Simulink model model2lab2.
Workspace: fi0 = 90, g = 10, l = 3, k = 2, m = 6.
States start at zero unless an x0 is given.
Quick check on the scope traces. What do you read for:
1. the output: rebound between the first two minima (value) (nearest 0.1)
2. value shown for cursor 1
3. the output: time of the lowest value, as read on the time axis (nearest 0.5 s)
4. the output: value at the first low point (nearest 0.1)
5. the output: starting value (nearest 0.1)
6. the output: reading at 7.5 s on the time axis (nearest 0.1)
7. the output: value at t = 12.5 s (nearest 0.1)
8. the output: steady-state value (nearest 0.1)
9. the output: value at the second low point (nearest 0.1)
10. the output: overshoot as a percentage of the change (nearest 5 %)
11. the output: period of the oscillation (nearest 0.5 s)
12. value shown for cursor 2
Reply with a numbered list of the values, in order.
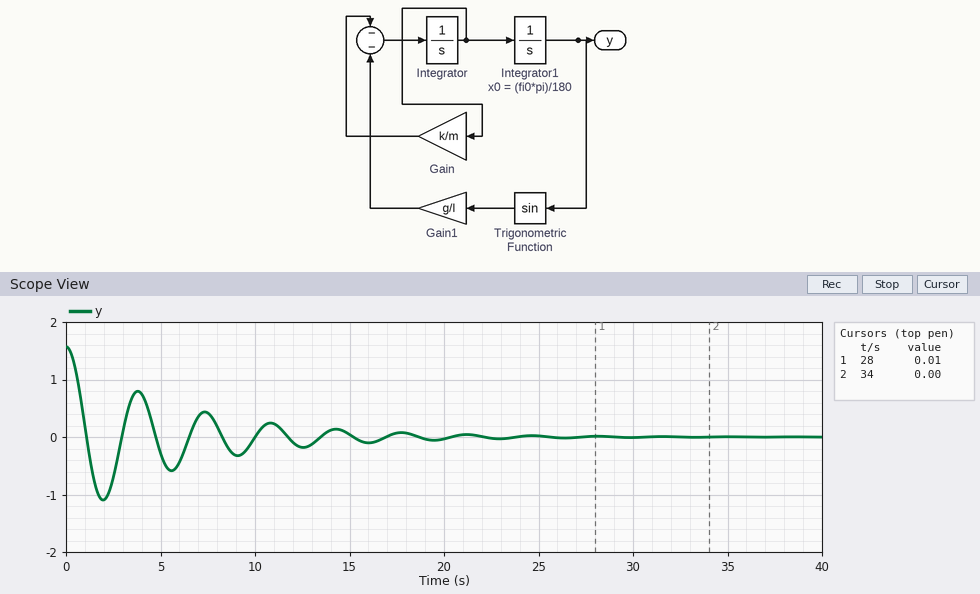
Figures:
1. 0.8
2. 0.01
3. 2.0 s
4. -1.1
5. 1.6
6. 0.4
7. -0.2
8. 0.0
9. -0.6
10. 70 %
11. 3.5 s
12. 0.00
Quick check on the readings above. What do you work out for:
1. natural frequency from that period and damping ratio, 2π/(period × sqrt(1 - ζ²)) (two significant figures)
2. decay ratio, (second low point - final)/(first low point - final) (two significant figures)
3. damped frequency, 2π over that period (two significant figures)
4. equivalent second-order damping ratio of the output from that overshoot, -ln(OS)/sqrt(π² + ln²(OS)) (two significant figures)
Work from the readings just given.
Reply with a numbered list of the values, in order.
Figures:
1. 1.8 rad/s
2. 0.55
3. 1.8 rad/s
4. 0.11
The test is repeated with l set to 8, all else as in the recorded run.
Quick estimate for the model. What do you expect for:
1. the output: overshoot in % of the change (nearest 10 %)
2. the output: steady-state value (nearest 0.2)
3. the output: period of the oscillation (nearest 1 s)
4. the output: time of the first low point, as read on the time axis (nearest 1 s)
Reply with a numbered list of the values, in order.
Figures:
1. 60 %
2. 0.0
3. 6 s
4. 3 s
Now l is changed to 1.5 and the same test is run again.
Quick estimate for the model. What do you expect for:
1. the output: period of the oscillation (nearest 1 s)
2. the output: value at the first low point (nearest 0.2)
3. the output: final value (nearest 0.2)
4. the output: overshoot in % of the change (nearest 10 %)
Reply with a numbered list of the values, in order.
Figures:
1. 3 s
2. -1.2
3. 0.0
4. 80 %
